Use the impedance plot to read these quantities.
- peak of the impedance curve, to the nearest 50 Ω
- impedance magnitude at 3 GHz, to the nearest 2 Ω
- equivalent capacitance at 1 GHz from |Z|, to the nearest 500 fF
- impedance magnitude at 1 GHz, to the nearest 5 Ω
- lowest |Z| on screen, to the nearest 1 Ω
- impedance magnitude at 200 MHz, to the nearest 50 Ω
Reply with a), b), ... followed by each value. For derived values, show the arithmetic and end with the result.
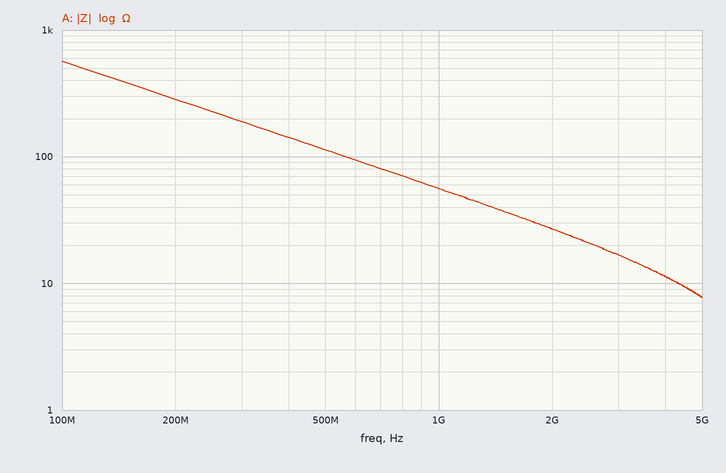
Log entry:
a) 550 Ω
b) 16 Ω
c) C = 1/(2π × 1 GHz × 55 Ω) ≈ 2.89 pF, so 3.0 pF to the nearest 500 fF
d) 55 Ω
e) 8 Ω
f) 300 Ω
